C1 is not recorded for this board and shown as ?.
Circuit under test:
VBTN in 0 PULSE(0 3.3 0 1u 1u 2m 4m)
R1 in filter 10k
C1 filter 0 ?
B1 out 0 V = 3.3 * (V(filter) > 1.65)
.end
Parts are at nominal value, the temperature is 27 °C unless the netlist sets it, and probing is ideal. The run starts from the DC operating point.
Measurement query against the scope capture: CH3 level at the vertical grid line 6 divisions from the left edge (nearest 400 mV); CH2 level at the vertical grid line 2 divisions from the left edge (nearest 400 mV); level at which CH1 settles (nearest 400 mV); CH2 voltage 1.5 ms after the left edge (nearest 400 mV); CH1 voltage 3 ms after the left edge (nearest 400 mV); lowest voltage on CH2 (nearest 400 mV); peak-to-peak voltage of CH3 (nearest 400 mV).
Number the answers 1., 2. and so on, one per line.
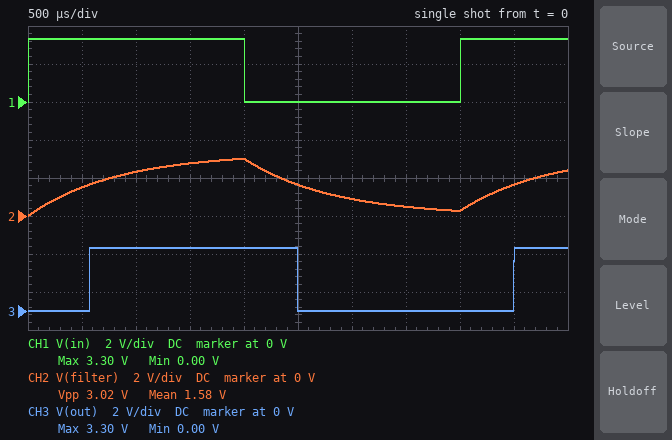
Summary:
1. 0 V
2. 2.4 V
3. 3.2 V
4. 2.8 V
5. 0 V
6. 0 V
7. 3.2 V
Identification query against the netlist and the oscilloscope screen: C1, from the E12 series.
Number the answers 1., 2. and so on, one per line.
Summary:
1. 82 nF
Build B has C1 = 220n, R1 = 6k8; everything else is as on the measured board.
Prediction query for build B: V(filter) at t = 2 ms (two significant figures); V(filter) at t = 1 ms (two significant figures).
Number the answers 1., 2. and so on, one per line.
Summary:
1. 2.4 V
2. 1.6 V
